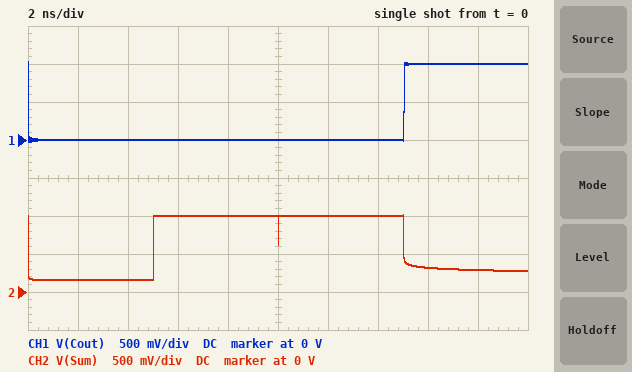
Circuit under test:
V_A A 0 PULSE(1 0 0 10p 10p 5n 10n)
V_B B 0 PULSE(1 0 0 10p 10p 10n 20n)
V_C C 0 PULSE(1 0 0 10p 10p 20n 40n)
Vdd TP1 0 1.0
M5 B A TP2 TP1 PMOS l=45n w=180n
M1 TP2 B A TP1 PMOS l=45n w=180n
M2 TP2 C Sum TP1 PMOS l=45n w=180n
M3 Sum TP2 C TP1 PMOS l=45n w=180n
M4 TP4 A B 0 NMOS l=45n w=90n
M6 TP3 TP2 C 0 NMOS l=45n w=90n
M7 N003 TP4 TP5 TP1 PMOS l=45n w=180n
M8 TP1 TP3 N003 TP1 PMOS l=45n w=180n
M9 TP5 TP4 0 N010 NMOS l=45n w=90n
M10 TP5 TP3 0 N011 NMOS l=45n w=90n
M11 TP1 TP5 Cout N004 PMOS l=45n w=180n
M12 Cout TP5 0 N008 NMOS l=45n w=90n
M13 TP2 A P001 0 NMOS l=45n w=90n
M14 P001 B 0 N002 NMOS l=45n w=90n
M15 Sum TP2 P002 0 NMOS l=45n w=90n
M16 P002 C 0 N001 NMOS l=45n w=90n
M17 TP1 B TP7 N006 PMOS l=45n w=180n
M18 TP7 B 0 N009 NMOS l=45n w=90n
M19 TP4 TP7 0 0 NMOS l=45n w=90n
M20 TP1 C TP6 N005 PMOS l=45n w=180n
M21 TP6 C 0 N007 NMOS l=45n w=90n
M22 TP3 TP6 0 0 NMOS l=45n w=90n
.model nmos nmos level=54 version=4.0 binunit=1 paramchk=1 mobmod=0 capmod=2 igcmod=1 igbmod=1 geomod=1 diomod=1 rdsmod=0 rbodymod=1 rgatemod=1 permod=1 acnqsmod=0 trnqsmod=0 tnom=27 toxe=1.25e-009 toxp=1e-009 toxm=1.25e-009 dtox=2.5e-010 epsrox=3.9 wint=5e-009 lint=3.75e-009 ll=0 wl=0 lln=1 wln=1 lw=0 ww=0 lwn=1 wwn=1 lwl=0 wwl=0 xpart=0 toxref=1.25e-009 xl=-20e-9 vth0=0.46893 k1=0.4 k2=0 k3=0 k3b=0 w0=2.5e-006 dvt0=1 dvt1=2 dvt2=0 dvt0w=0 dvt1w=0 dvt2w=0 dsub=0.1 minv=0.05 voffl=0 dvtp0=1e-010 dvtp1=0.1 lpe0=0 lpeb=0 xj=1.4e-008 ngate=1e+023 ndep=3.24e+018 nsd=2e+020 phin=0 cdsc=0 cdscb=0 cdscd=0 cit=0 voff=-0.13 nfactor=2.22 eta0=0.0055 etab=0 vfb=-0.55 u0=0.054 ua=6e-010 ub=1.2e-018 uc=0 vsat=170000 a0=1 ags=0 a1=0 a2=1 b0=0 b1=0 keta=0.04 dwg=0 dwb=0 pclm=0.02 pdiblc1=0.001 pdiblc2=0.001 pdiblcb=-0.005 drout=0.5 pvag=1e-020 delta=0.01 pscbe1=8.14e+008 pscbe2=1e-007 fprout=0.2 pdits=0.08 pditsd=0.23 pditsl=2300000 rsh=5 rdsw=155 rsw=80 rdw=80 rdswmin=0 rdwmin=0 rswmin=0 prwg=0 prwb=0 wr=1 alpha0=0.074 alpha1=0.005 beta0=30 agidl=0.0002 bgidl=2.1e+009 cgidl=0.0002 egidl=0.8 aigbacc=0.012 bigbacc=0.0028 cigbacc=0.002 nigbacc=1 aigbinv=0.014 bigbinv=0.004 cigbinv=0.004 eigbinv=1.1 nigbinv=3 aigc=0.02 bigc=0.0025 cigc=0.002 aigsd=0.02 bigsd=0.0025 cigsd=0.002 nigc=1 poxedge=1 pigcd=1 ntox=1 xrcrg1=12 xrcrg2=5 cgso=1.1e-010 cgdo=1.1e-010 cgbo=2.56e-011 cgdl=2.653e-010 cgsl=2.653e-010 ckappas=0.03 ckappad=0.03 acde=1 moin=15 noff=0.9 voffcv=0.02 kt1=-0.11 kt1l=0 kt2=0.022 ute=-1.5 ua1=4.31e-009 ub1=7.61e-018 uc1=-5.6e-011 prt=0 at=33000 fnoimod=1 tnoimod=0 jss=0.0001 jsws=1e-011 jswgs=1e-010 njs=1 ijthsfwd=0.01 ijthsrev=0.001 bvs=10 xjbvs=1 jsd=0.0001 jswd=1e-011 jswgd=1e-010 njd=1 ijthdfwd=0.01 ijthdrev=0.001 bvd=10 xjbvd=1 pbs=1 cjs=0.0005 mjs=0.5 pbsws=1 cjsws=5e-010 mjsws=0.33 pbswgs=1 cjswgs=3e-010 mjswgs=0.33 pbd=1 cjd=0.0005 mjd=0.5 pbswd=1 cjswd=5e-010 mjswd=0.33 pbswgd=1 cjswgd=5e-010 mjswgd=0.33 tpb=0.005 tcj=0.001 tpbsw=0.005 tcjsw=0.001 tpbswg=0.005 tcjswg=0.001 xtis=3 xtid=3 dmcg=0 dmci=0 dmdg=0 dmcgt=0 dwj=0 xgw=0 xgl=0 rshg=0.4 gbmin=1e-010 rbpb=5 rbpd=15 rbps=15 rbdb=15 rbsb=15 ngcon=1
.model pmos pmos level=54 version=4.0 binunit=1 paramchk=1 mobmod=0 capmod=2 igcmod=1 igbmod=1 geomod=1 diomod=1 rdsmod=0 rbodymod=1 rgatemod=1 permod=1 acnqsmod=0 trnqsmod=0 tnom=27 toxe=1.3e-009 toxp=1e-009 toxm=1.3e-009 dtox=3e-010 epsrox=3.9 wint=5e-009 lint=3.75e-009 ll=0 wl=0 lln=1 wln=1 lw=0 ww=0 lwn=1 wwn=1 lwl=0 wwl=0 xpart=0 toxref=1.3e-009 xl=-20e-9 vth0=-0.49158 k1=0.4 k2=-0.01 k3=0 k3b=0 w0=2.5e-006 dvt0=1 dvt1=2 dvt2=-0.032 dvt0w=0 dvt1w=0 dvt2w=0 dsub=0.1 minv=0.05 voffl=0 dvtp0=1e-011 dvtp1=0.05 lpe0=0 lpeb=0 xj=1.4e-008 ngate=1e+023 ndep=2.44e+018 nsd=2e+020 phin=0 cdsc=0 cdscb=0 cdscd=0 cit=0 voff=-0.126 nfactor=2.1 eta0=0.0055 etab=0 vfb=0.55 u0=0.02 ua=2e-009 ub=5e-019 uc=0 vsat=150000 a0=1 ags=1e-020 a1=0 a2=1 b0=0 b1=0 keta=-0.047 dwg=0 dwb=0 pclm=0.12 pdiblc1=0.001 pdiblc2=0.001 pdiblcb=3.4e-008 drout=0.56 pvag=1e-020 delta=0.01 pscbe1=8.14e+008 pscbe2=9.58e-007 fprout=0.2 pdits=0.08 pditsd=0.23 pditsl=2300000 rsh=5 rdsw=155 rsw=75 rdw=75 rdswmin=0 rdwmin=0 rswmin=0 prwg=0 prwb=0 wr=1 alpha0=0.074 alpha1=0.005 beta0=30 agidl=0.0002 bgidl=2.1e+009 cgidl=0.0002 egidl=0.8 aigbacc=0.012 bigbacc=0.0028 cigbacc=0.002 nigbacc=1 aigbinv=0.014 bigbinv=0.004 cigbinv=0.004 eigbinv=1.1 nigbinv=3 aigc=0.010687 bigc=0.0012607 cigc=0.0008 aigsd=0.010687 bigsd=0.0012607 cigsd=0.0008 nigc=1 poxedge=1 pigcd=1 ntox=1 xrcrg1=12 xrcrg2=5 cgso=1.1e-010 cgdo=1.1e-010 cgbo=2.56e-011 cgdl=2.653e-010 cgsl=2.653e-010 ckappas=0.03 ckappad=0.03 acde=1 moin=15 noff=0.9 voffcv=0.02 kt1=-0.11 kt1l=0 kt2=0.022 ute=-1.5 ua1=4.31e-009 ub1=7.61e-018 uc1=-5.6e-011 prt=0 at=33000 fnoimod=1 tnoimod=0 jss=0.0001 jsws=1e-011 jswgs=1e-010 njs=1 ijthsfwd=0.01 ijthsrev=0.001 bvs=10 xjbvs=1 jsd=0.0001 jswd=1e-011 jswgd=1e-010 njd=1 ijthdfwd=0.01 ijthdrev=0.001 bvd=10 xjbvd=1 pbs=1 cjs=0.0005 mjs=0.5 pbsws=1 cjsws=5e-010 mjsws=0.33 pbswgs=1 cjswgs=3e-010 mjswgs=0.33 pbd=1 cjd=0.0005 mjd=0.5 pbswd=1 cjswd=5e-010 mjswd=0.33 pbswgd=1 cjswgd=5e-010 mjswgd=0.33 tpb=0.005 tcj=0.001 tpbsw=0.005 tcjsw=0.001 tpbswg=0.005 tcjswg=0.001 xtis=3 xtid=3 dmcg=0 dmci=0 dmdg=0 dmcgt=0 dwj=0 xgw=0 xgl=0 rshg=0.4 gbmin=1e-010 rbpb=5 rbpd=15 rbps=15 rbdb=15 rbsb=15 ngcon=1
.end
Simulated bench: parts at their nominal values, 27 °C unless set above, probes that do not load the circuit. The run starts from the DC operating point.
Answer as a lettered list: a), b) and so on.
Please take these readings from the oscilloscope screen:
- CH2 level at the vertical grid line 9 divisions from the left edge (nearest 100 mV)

a) 300 mV
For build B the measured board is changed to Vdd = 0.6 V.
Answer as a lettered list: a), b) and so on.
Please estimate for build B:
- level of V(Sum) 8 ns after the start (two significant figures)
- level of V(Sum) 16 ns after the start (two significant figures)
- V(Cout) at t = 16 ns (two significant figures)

a) 1.0 V
b) 270 mV
c) 600 mV
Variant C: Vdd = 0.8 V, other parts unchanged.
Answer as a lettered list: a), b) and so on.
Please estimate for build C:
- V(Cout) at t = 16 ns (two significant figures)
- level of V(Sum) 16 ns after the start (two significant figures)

a) 800 mV
b) 290 mV
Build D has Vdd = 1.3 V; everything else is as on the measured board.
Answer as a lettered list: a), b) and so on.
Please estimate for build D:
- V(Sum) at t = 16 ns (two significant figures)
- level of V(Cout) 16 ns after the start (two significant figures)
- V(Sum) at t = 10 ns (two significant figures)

a) 350 mV
b) 1.3 V
c) 1.0 V
